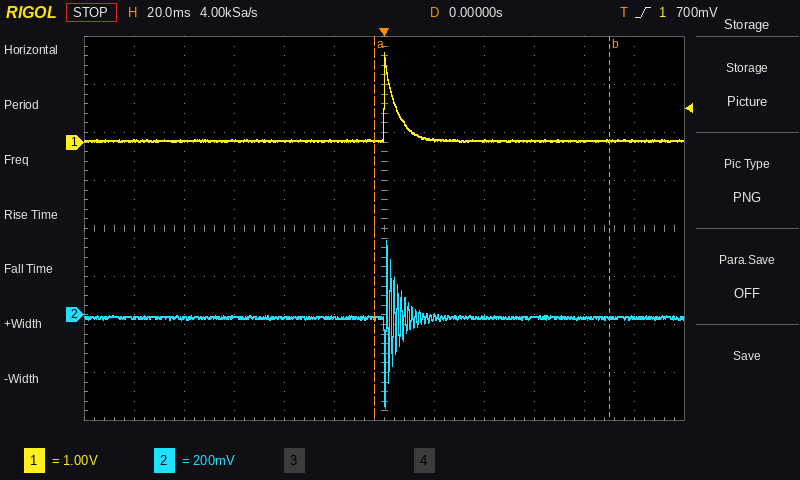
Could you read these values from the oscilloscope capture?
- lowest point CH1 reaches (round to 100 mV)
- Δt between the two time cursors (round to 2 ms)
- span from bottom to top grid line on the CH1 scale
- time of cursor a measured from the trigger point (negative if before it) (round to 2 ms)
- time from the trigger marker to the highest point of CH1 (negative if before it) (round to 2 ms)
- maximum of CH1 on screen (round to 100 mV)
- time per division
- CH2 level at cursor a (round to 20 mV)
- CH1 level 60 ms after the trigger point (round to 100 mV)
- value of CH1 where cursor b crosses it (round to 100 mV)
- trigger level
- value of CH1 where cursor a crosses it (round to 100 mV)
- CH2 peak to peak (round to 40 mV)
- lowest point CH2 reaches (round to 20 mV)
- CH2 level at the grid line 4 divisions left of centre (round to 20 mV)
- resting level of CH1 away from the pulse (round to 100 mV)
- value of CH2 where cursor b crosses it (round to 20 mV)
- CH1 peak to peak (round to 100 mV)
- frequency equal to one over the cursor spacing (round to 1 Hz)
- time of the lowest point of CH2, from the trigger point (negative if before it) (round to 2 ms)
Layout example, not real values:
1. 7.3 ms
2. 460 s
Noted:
1. 0.0 V
2. 94 ms
3. 8 V
4. -4 ms
5. 0 ms
6. 1.9 V
7. 20 ms
8. -20 mV
9. 0.0 V
10. 0.0 V
11. 700 mV
12. 0.0 V
13. 680 mV
14. -380 mV
15. -20 mV
16. 0.0 V
17. -20 mV
18. 1.9 V
19. 11 Hz
20. 0 ms
